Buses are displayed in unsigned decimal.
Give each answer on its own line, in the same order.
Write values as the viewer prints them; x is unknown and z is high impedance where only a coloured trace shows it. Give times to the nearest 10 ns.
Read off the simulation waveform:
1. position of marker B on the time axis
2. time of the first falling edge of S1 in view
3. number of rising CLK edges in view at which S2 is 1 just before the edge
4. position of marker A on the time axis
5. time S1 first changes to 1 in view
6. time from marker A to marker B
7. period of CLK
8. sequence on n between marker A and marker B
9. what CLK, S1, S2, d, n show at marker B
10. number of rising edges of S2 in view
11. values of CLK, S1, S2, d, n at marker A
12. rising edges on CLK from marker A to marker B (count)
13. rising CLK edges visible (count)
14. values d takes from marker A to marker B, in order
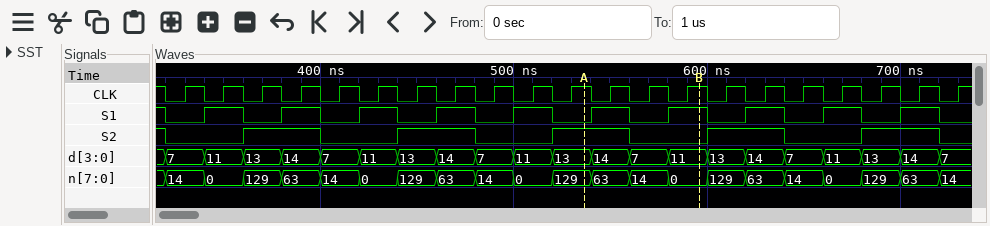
600 ns
320 ns
10
540 ns
340 ns
60 ns
20 ns
129, 63, 14, 0
CLK=1, S1=1, S2=0, d=11, n=0
5
CLK=1, S1=0, S2=1, d=13, n=129
3
21
13, 14, 7, 11
